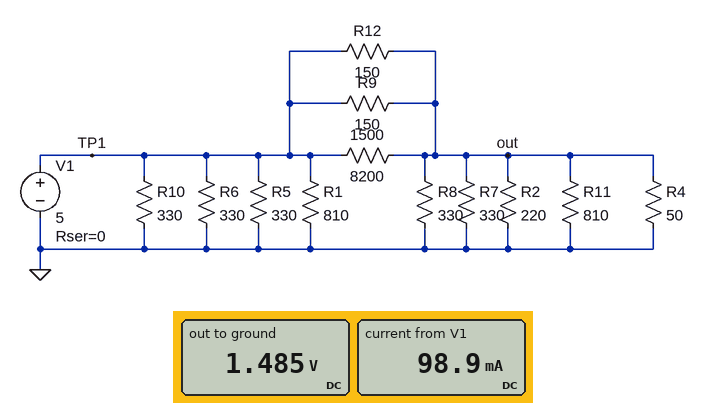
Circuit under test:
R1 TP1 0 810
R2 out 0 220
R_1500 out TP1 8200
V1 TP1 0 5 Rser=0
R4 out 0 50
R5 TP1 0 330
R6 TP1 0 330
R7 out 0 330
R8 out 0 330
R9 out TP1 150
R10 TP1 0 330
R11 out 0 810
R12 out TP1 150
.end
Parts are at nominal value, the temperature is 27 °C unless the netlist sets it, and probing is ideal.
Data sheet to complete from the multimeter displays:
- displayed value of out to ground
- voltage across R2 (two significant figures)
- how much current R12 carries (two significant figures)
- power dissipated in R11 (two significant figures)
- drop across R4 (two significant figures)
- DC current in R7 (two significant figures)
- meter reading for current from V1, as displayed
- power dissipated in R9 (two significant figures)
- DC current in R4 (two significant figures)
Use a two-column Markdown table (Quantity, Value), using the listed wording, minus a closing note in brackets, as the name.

| Quantity | Value |
|---|---|
| displayed value of out to ground | 1.485 V |
| voltage across R2 | 1.5 V |
| how much current R12 carries | 23 mA |
| power dissipated in R11 | 2.7 mW |
| drop across R4 | 1.5 V |
| DC current in R7 | 4.5 mA |
| meter reading for current from V1, as displayed | 98.9 mA |
| power dissipated in R9 | 82 mW |
| DC current in R4 | 30 mA |
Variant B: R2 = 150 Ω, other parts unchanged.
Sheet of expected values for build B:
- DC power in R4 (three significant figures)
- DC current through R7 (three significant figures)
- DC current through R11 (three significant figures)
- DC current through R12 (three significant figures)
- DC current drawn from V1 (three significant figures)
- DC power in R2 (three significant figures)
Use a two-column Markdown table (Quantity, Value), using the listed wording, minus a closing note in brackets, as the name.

| Quantity | Value |
|---|---|
| DC power in R4 | 40.3 mW |
| DC current through R7 | 4.30 mA |
| DC current through R11 | 1.75 mA |
| DC current through R12 | 23.9 mA |
| DC current drawn from V1 | 99.8 mA |
| DC power in R2 | 13.4 mW |
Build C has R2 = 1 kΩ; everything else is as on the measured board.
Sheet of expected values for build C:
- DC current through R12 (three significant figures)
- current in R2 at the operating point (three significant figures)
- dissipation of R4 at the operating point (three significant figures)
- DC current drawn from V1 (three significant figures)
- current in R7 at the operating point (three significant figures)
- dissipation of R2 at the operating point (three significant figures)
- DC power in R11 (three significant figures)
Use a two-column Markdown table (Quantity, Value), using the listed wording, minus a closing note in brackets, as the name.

| Quantity | Value |
|---|---|
| DC current through R12 | 22.6 mA |
| current in R2 at the operating point | 1.61 mA |
| dissipation of R4 at the operating point | 51.9 mW |
| DC current drawn from V1 | 97.2 mA |
| current in R7 at the operating point | 4.88 mA |
| dissipation of R2 at the operating point | 2.60 mW |
| DC power in R11 | 3.21 mW |
